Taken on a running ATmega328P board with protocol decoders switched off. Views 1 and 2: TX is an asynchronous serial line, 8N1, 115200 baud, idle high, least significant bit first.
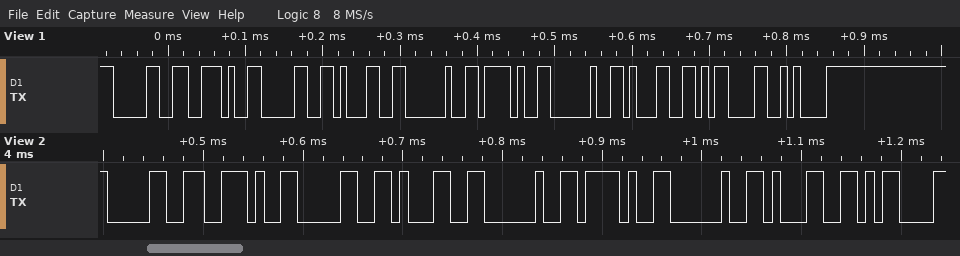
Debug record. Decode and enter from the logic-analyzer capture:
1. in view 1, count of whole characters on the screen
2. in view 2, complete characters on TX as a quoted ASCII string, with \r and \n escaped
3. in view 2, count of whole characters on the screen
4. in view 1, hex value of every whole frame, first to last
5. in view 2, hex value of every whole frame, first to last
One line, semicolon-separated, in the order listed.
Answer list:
10; "0.01 / 1\r"; 9; 0x30 0x2E 0x30 0x31 0x20 0x2F 0x20 0x31 0x0D 0x0A; 30 2E 30 31 20 2F 20 31 0D
